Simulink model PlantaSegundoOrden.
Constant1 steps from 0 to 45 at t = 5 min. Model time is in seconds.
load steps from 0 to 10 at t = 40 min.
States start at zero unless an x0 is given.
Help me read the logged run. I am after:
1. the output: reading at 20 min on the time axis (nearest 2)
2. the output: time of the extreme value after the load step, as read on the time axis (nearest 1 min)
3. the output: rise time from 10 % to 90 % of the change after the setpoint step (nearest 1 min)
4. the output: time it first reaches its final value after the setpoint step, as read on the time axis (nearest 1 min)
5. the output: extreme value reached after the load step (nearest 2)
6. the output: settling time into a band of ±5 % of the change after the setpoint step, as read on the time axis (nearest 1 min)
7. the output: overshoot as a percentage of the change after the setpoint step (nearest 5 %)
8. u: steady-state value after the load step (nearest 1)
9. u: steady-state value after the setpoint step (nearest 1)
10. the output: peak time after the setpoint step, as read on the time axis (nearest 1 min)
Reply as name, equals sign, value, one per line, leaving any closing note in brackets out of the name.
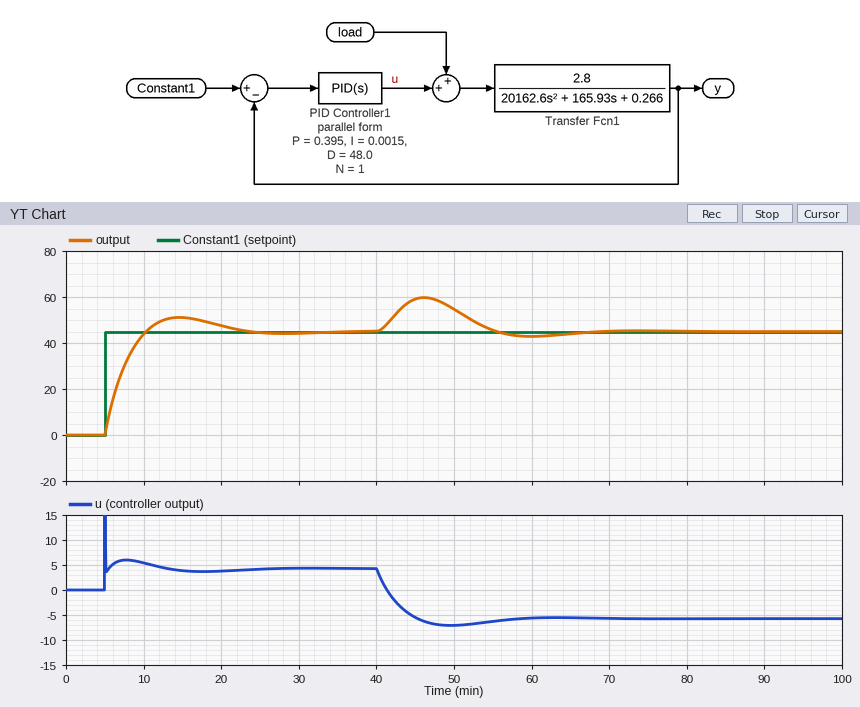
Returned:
the output: reading at 20 min on the time axis = 48
the output: time of the extreme value after the load step, as read on the time axis = 46 min
the output: rise time from 10 % to 90 % of the change after the setpoint step = 4 min
the output: time it first reaches its final value after the setpoint step, as read on the time axis = 10 min
the output: extreme value reached after the load step = 60
the output: settling time into a band of ±5 % of the change after the setpoint step, as read on the time axis = 20 min
the output: overshoot as a percentage of the change after the setpoint step = 15 %
u: steady-state value after the load step = -6
u: steady-state value after the setpoint step = 4
the output: peak time after the setpoint step, as read on the time axis = 15 min
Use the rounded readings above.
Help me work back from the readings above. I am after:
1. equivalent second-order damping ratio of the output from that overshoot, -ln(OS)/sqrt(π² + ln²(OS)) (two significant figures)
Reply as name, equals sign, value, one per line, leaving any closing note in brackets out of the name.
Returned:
equivalent second-order damping ratio of the output from that overshoot, -ln(OS)/sqrt(π² + ln²(OS)) = 0.52
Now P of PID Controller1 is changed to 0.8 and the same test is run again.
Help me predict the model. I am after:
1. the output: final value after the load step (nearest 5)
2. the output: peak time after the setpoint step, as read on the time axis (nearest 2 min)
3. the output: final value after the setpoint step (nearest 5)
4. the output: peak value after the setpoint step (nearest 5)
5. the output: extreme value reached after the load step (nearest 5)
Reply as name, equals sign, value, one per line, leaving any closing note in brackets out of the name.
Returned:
the output: final value after the load step = 45
the output: peak time after the setpoint step, as read on the time axis = 10 min
the output: final value after the setpoint step = 45
the output: peak value after the setpoint step = 50
the output: extreme value reached after the load step = 55
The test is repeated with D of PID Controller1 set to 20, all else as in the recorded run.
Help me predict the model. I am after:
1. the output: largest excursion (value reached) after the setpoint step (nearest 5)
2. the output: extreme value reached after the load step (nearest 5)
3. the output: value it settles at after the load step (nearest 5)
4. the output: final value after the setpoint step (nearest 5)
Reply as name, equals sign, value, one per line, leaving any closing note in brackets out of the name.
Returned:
the output: largest excursion (value reached) after the setpoint step = 55
the output: extreme value reached after the load step = 60
the output: value it settles at after the load step = 45
the output: final value after the setpoint step = 45
